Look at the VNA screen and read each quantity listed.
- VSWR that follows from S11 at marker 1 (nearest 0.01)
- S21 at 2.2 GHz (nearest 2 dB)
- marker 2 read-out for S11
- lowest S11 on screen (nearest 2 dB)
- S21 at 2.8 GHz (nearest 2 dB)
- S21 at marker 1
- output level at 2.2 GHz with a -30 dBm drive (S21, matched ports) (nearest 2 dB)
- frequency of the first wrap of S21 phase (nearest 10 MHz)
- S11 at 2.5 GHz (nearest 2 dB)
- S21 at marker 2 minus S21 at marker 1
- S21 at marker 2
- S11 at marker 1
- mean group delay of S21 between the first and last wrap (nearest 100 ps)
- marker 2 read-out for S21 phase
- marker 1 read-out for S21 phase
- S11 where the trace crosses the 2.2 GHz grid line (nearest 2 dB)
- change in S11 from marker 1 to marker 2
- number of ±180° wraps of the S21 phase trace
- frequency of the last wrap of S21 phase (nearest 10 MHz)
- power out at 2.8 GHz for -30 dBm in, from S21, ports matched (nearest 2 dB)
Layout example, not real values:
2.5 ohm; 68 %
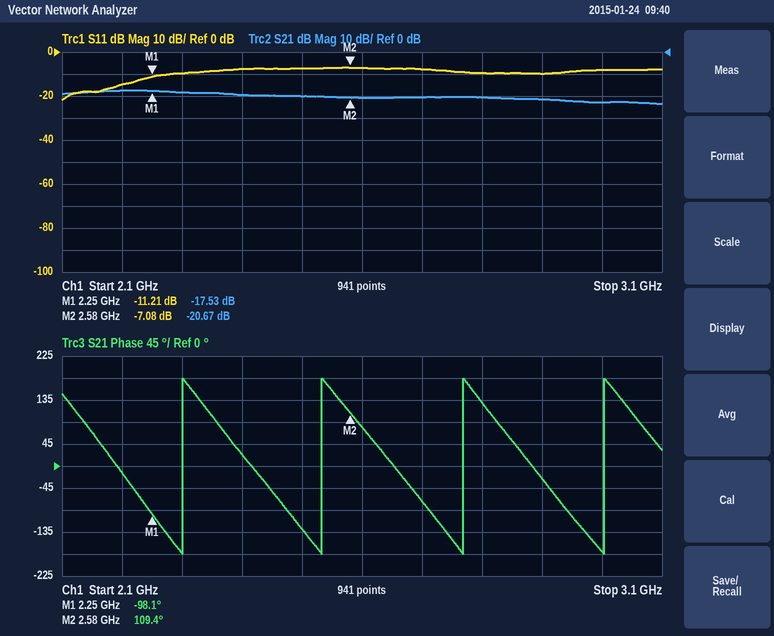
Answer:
1.76; -18 dB; -7.08 dB; -22 dB; -20 dB; -17.53 dB; -48 dBm; 2.30 GHz; -8 dB; -3.14 dB; -20.67 dB; -11.21 dB; 4.3 ns; 109.4°; -98.1°; -14 dB; 4.13 dB; 4; 3.00 GHz; -50 dBm
